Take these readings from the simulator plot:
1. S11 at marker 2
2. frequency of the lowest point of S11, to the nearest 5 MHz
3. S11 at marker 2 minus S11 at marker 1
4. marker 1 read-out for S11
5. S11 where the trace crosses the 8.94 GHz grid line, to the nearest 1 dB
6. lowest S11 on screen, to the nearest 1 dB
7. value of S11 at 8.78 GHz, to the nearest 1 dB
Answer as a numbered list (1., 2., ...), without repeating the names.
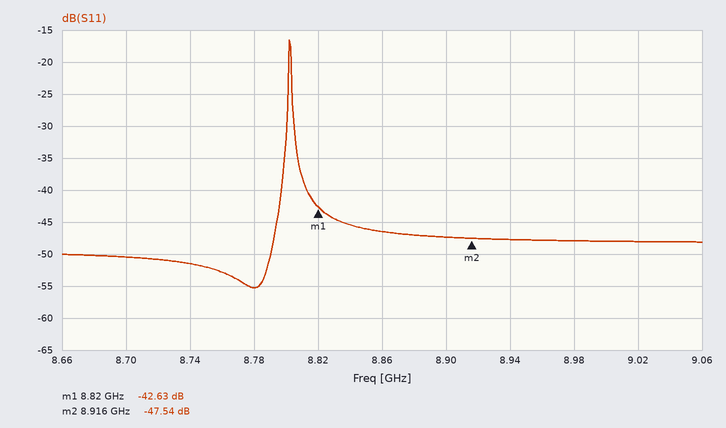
1. -47.54 dB
2. 8.780 GHz
3. -4.91 dB
4. -42.63 dB
5. -48 dB
6. -55 dB
7. -55 dB
